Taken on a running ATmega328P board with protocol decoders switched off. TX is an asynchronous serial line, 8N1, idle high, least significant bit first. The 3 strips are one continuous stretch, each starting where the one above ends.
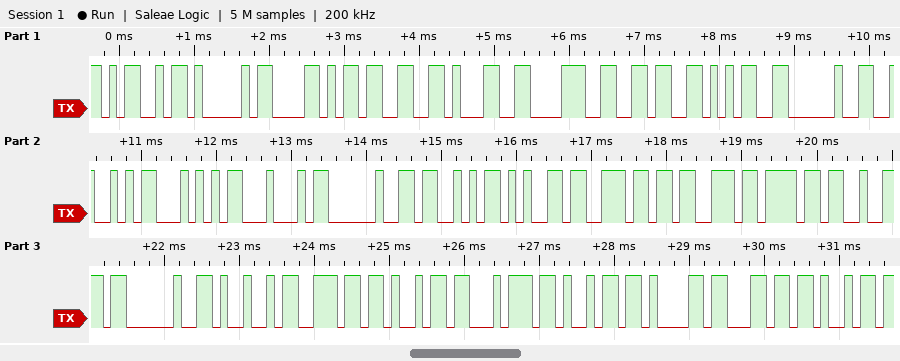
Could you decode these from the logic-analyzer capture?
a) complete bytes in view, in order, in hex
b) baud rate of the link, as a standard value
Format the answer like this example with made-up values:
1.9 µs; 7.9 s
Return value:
4D 41 58 33 31 38 36 35 20 52 54 44 20 53 65 6E 73 6F 72 20 49 6E 69 74 69 61 6C 69; 9600 baud
